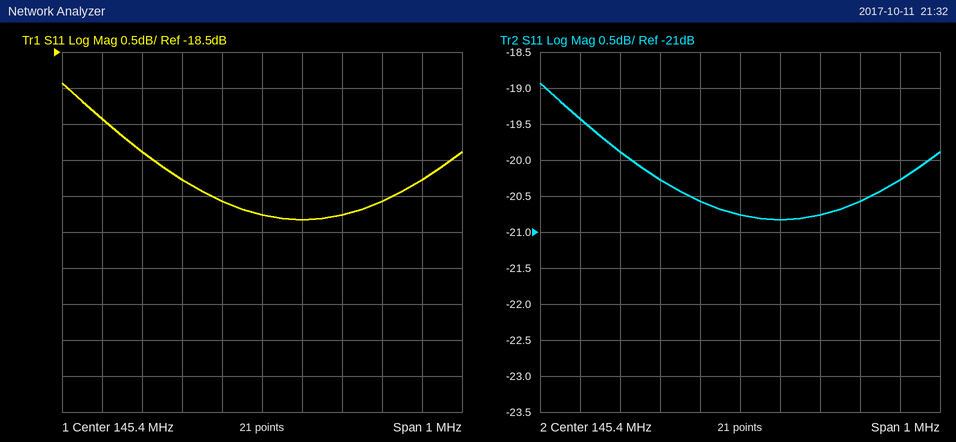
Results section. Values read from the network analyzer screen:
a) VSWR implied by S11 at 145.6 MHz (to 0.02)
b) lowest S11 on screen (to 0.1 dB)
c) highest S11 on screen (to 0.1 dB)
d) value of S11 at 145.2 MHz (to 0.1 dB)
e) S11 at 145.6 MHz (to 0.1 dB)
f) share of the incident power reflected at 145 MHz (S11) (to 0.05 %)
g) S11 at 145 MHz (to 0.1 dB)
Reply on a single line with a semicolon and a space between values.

1.20; -20.8 dB; -18.9 dB; -20.3 dB; -20.8 dB; 1.15 %; -19.4 dB
